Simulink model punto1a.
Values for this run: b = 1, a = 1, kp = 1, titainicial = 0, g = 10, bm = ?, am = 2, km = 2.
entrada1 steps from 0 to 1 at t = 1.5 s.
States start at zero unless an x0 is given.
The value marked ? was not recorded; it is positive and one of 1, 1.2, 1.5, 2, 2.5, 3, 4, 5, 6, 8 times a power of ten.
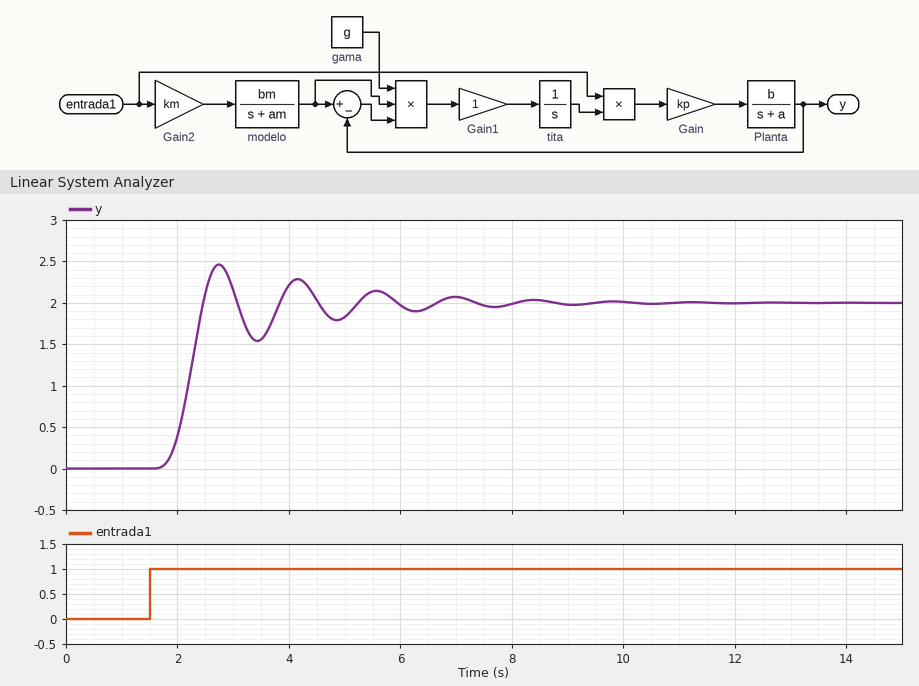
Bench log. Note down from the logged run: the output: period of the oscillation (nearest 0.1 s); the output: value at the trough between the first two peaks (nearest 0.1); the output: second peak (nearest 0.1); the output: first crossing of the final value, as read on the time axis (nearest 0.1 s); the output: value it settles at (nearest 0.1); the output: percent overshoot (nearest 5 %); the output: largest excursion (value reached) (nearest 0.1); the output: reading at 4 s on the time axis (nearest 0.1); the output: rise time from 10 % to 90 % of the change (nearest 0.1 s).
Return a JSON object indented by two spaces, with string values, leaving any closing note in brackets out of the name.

{
  "the output: period of the oscillation": "1.4 s",
  "the output: value at the trough between the first two peaks": "1.5",
  "the output: second peak": "2.3",
  "the output: first crossing of the final value, as read on the time axis": "2.5 s",
  "the output: value it settles at": "2.0",
  "the output: percent overshoot": "25 %",
  "the output: largest excursion (value reached)": "2.5",
  "the output: reading at 4 s on the time axis": "2.2",
  "the output: rise time from 10 % to 90 % of the change": "0.5 s"
}
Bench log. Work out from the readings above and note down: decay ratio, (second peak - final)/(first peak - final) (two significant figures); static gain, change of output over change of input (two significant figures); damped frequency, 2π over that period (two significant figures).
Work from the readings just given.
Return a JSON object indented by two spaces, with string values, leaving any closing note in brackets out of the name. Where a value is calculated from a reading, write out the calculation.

{
  "decay ratio, (second peak - final)/(first peak - final)": "(2.3 - 2) / (2.5 - 2) = 0.60",
  "static gain, change of output over change of input": "(2 - 0) / (1 - 0) = 2.0",
  "damped frequency, 2π over that period": "2π / 1.4 = 4.5 rad/s"
}
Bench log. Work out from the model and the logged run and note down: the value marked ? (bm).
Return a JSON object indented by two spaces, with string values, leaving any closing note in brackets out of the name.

{
  "the value marked ?": "2"
}
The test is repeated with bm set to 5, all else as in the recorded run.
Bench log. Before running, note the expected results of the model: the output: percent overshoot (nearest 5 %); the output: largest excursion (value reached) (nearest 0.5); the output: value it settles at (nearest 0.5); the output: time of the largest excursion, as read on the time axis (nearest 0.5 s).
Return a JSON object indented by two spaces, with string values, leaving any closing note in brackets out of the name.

{
  "the output: percent overshoot": "15 %",
  "the output: largest excursion (value reached)": "5.5",
  "the output: value it settles at": "5.0",
  "the output: time of the largest excursion, as read on the time axis": "3.5 s"
}
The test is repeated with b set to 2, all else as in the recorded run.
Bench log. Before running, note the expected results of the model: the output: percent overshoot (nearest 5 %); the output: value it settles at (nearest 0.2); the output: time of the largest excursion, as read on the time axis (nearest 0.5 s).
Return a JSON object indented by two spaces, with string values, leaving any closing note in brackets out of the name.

{
  "the output: percent overshoot": "15 %",
  "the output: value it settles at": "2.0",
  "the output: time of the largest excursion, as read on the time axis": "3.5 s"
}
